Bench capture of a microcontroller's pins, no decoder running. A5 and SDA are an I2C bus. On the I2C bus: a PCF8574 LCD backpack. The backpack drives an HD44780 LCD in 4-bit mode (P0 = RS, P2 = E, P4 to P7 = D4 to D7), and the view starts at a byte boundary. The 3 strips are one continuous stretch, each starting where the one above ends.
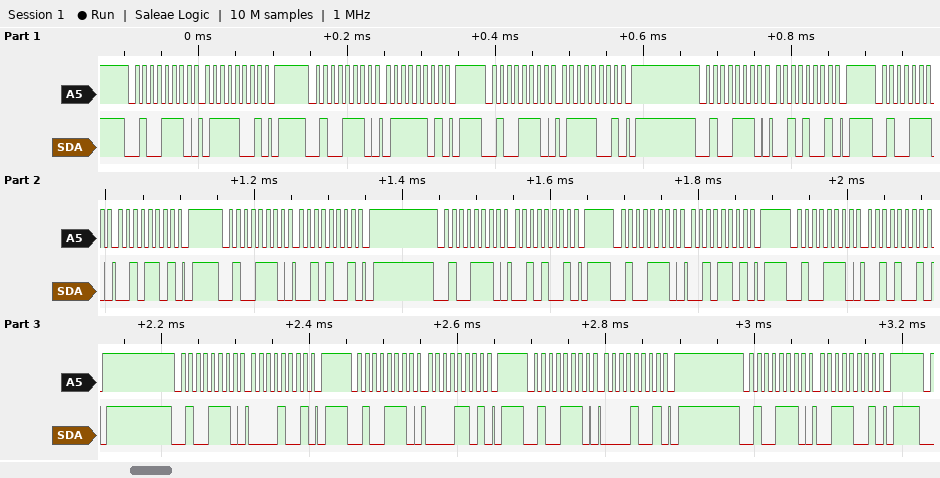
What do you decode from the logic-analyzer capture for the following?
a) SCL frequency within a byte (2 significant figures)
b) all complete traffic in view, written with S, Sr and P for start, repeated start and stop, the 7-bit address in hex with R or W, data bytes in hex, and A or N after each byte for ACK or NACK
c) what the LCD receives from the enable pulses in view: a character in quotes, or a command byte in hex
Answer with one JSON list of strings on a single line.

["100 kHz", "S 27W A 79 A P S 27W A 7D A P S 27W A 79 A P S 27W A 29 A P S 27W A 2D A P S 27W A 29 A P S 27W A 29 A P S 27W A 2D A P S 27W A 29 A P S 27W A 09 A P S 27W A 0D A P S 27W A 09 A P S 27W A 39 A P", "'r' ' '"]
